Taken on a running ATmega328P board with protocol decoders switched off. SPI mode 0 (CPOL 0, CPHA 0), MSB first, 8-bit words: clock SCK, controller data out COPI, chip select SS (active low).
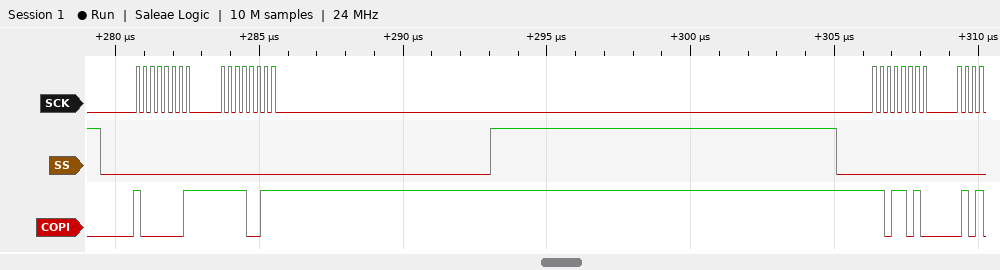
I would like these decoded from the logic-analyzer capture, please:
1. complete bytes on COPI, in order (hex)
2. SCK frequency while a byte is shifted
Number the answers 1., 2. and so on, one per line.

1. 81 F3 DA
2. 4 MHz
